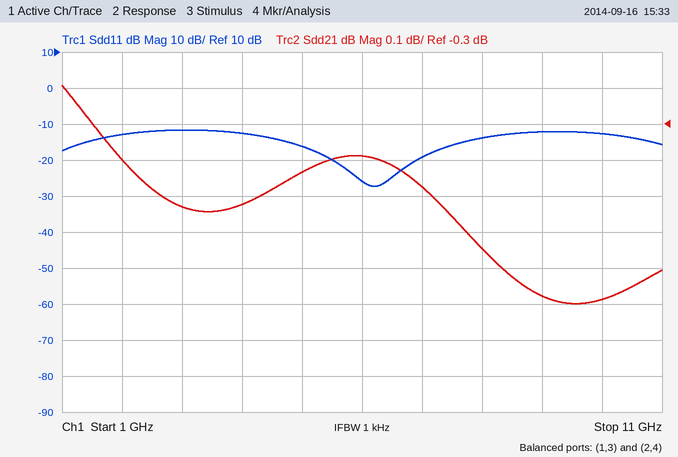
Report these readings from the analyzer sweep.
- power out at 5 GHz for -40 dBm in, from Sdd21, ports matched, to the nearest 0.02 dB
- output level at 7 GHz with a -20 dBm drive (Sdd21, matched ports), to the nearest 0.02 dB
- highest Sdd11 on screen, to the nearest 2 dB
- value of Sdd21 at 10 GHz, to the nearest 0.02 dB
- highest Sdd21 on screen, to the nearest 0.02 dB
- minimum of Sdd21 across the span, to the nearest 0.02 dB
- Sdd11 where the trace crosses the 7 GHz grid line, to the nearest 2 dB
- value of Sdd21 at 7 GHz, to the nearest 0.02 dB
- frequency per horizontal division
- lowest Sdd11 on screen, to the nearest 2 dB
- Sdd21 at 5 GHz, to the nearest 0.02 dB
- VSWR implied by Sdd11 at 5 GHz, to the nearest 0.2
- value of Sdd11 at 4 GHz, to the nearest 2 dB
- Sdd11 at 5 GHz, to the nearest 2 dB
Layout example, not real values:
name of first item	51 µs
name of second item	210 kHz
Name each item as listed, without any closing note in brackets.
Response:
power out at 5 GHz for -40 dBm in, from Sdd21, ports matched, to the nearest 0.02 dB	-40.44 dBm
output level at 7 GHz with a -20 dBm drive (Sdd21, matched ports), to the nearest 0.02 dB	-20.48 dBm
highest Sdd11 on screen, to the nearest 2 dB	-12 dB
value of Sdd21 at 10 GHz, to the nearest 0.02 dB	-0.78 dB
highest Sdd21 on screen, to the nearest 0.02 dB	-0.20 dB
minimum of Sdd21 across the span, to the nearest 0.02 dB	-0.80 dB
Sdd11 where the trace crosses the 7 GHz grid line, to the nearest 2 dB	-20 dB
value of Sdd21 at 7 GHz, to the nearest 0.02 dB	-0.48 dB
frequency per horizontal division	1 GHz
lowest Sdd11 on screen, to the nearest 2 dB	-28 dB
Sdd21 at 5 GHz, to the nearest 0.02 dB	-0.44 dB
VSWR implied by Sdd11 at 5 GHz, to the nearest 0.2	1.4
value of Sdd11 at 4 GHz, to the nearest 2 dB	-12 dB
Sdd11 at 5 GHz, to the nearest 2 dB	-16 dB
